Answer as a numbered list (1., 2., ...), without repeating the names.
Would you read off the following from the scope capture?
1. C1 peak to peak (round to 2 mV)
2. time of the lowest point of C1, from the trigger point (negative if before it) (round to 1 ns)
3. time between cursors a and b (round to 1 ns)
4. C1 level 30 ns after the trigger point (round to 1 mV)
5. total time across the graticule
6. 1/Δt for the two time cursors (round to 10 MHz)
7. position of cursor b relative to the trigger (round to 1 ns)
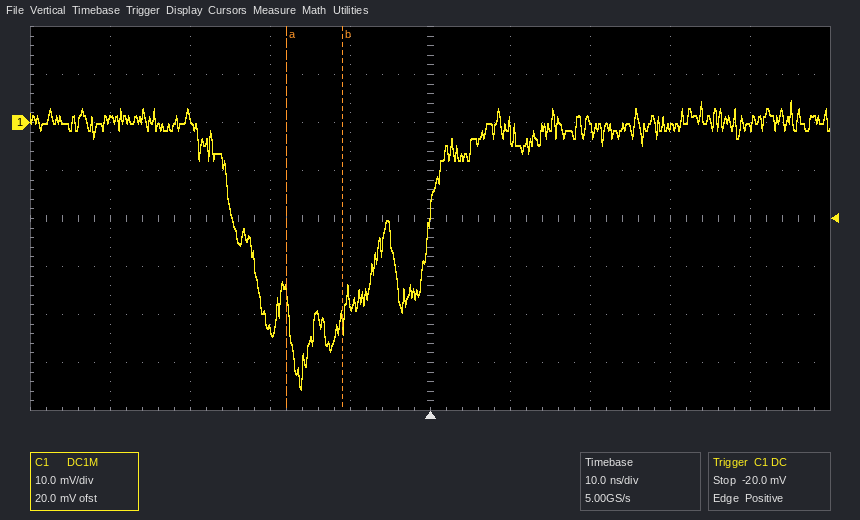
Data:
1. 60 mV
2. -16 ns
3. 7 ns
4. -1 mV
5. 100 ns
6. 140 MHz
7. -11 ns
